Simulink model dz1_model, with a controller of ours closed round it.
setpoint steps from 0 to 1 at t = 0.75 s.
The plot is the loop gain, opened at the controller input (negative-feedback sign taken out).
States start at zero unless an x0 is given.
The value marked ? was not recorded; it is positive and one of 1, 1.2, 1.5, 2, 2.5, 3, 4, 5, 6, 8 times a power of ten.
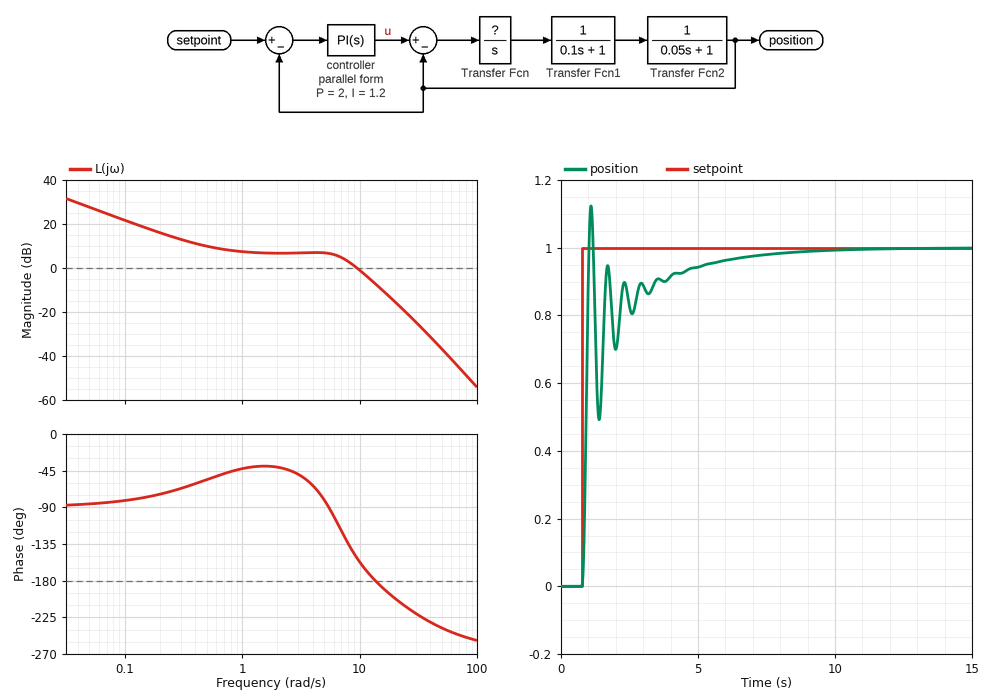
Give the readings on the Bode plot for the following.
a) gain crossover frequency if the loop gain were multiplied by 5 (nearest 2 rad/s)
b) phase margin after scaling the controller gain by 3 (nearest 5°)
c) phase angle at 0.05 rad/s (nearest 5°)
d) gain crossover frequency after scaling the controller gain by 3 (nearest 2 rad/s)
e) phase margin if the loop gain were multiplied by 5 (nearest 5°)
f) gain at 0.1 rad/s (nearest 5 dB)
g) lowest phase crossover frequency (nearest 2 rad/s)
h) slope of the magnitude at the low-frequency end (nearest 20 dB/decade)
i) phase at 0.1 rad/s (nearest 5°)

18 rad/s
-5°
-85°
16 rad/s
-20°
20 dB
14 rad/s
-20 dB/decade
-80°
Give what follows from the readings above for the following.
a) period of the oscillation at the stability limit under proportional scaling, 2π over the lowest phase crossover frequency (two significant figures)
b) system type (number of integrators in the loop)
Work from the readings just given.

0.45 s
1
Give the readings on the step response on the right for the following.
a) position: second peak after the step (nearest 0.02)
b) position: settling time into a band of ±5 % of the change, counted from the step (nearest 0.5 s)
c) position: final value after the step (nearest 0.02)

0.94
4.5 s
1.00
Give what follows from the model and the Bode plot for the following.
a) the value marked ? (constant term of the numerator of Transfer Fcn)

5
